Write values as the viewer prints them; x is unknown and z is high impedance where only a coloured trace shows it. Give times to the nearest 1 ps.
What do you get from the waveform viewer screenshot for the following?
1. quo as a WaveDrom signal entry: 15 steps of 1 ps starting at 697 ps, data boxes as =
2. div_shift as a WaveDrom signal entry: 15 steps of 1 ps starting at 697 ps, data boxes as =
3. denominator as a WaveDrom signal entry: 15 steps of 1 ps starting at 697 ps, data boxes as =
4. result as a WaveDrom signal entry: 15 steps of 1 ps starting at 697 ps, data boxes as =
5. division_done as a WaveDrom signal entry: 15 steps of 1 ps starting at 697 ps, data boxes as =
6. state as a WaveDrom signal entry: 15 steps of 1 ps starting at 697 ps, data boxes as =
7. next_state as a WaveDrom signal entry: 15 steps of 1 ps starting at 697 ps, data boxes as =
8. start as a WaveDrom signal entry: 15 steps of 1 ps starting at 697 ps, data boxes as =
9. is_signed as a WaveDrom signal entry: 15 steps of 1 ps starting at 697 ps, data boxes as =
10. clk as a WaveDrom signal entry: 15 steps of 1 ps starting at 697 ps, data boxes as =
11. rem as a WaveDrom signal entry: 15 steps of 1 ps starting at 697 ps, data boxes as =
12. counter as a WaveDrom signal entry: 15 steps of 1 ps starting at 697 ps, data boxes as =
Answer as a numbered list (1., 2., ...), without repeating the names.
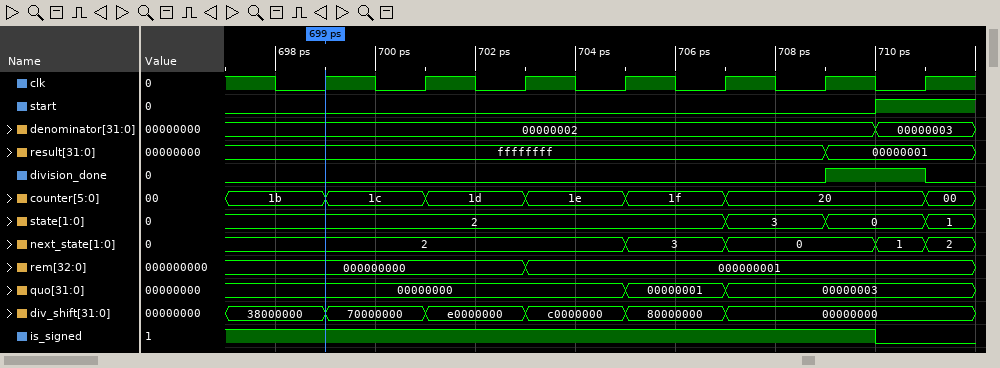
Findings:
1. {name: 'quo', wave: '=.......=.=....', data: '00000000 00000001 00000003'}
2. {name: 'div_shift', wave: '=.=.=.=.=.=....', data: '38000000 70000000 e0000000 c0000000 80000000 00000000'}
3. {name: 'denominator', wave: '=............=.', data: '00000002 00000003'}
4. {name: 'result', wave: '=...........=..', data: 'ffffffff 00000001'}
5. {name: 'division_done', wave: '0...........1.0'}
6. {name: 'state', wave: '=.........=.=.=', data: '2 3 0 1'}
7. {name: 'next_state', wave: '=.......=.=..==', data: '2 3 0 1 2'}
8. {name: 'start', wave: '0............1.'}
9. {name: 'is_signed', wave: '1............0.'}
10. {name: 'clk', wave: '101010101010101'}
11. {name: 'rem', wave: '=.....=........', data: '000000000 000000001'}
12. {name: 'counter', wave: '=.=.=.=.=.=...=', data: '1b 1c 1d 1e 1f 20 00'}
